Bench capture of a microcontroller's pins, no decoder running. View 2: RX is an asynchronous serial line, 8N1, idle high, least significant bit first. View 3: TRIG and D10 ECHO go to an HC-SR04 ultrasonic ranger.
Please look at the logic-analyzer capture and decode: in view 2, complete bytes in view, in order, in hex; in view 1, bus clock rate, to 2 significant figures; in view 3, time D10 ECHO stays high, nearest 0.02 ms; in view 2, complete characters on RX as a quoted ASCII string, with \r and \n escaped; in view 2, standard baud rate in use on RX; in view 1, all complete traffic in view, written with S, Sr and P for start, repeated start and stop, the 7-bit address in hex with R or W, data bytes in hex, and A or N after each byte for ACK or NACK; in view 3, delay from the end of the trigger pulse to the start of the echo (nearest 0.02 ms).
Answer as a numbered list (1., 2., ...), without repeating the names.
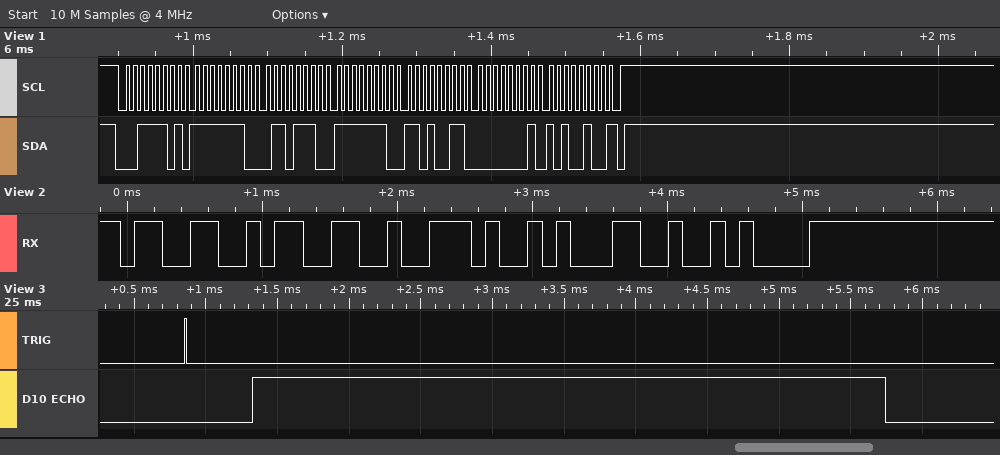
1. 0x33 0x33 0x2E 0x31 0x0A
2. 100 kHz
3. 4.42 ms
4. "33.1\n"
5. 9600 baud
6. S 1ER A FE A 6E A FE A D3 A 01 A A4 N P
7. 0.46 ms
